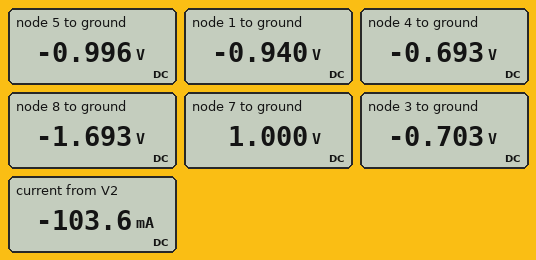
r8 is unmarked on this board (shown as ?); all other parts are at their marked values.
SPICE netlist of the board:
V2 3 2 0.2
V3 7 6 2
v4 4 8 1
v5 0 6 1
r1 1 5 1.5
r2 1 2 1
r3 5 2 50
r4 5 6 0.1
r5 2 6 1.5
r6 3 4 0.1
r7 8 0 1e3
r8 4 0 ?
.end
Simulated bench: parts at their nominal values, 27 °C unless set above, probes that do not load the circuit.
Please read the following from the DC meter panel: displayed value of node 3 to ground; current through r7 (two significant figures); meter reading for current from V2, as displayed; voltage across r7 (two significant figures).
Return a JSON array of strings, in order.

["-0.703 V", "1.7 mA", "-103.6 mA", "1.7 V"]
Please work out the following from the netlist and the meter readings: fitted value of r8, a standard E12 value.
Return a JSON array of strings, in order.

["6.8 Ω"]
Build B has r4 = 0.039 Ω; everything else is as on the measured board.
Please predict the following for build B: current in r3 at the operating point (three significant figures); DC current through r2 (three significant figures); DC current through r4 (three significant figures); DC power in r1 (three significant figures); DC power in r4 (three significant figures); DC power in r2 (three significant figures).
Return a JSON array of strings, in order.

["1.89 mA", "37.8 mA", "39.7 mA", "2.14 mW", "61.4 µW", "1.43 mW"]
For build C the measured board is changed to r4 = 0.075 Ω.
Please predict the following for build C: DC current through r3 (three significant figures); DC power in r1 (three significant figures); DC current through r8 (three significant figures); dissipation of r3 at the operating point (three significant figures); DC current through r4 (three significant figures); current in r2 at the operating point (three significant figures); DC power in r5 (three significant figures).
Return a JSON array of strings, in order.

["1.87 mA", "2.10 mW", "102 mA", "175 µW", "39.3 mA", "37.4 mA", "6.21 mW"]
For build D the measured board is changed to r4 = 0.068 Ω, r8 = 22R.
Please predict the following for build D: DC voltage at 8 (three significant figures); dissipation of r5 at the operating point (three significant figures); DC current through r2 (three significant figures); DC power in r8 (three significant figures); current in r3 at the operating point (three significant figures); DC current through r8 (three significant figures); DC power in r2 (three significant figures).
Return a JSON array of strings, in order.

["-1.76 V", "765 µW", "13.2 mA", "26.4 mW", "659 µA", "34.7 mA", "174 µW"]
